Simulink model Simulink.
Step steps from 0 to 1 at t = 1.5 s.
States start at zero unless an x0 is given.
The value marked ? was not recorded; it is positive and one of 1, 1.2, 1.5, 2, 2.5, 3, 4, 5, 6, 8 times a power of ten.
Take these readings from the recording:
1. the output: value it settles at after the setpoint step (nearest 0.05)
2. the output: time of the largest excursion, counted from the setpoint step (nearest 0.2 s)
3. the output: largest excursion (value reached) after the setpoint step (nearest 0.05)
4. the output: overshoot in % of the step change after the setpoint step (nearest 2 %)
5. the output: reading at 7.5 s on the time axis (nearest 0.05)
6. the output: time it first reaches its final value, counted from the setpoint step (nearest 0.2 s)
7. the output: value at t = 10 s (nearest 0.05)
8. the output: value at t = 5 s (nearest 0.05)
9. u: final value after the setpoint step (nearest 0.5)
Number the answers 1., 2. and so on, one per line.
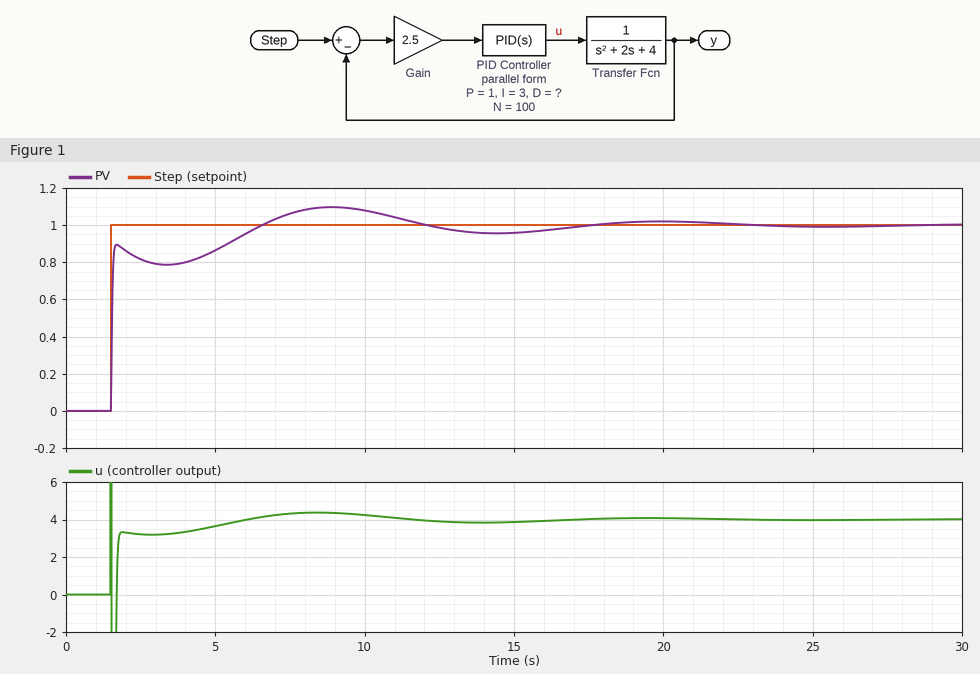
1. 1.00
2. 7.4 s
3. 1.10
4. 10 %
5. 1.05
6. 5.0 s
7. 1.10
8. 0.85
9. 4.0
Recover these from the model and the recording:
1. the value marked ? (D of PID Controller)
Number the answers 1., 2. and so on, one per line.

1. 8
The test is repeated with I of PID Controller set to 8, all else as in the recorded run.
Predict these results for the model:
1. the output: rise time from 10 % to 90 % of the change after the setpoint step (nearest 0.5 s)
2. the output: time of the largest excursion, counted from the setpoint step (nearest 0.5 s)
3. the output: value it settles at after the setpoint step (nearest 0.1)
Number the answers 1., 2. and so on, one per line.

1. 2.0 s
2. 4.5 s
3. 1.0
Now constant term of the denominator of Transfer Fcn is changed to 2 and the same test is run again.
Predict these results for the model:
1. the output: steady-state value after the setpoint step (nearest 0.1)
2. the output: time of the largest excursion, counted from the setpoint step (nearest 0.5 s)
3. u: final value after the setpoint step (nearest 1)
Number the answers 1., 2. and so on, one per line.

1. 1.0
2. 7.0 s
3. 2
